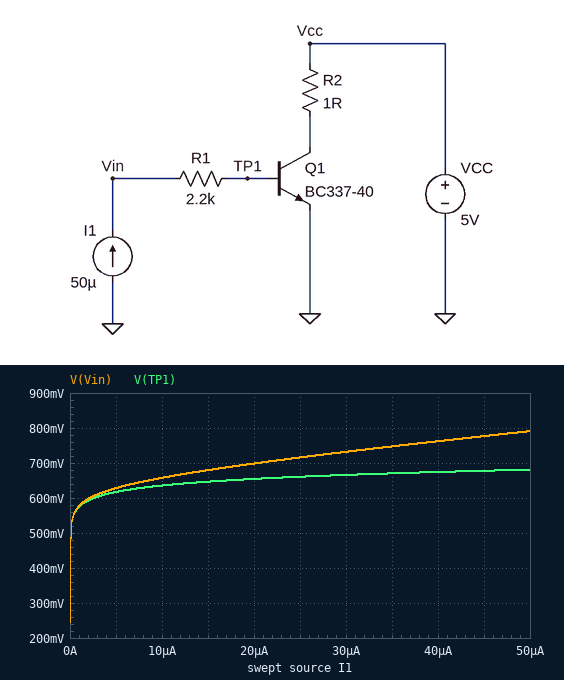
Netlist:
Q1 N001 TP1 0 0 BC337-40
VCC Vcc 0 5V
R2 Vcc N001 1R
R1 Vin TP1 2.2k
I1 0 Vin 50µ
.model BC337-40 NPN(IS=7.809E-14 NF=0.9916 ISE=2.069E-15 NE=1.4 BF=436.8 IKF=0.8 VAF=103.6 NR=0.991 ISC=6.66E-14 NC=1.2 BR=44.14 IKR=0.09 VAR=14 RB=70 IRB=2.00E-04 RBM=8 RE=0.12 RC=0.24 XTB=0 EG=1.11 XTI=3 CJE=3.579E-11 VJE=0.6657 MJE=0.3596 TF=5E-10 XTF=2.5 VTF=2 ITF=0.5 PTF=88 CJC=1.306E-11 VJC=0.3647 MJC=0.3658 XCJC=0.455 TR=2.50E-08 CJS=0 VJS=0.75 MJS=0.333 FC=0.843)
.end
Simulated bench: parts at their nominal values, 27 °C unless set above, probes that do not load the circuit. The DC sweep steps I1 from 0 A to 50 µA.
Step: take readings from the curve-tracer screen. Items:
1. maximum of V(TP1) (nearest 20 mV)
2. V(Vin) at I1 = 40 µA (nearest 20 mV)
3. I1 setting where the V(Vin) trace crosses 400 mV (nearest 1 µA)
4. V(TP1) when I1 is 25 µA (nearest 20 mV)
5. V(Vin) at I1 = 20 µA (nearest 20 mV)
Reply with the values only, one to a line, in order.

680 mV
760 mV
0 A
660 mV
700 mV
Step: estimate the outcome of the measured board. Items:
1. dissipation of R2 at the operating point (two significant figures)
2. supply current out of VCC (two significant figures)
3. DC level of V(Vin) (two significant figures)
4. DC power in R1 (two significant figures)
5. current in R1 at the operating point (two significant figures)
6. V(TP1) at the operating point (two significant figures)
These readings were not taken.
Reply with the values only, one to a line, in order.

440 µW
21 mA
790 mV
5.5 µW
50 µA
680 mV
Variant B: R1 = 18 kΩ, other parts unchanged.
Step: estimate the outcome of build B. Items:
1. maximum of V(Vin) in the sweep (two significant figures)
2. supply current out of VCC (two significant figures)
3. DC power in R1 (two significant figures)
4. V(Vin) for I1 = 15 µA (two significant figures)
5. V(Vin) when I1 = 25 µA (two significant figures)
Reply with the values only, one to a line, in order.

1.6 V
21 mA
45 µW
920 mV
1.1 V
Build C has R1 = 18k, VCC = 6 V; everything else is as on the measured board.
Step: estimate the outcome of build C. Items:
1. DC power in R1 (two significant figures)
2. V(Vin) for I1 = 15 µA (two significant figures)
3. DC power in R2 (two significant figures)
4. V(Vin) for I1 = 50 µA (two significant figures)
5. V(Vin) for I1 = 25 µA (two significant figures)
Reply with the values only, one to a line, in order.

45 µW
920 mV
450 µW
1.6 V
1.1 V
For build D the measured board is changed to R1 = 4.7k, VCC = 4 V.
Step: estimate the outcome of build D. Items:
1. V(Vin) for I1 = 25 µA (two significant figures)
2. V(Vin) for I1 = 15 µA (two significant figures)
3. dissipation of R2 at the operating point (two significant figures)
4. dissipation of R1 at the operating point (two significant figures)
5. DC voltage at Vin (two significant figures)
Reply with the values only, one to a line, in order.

780 mV
720 mV
430 µW
12 µW
920 mV
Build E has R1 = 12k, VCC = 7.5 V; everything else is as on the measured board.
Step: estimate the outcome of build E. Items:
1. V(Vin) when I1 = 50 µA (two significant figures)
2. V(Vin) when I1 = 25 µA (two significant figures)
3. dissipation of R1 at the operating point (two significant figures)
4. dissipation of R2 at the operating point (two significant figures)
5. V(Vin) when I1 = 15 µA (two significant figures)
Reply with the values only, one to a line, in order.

1.3 V
960 mV
30 µW
460 µW
830 mV
